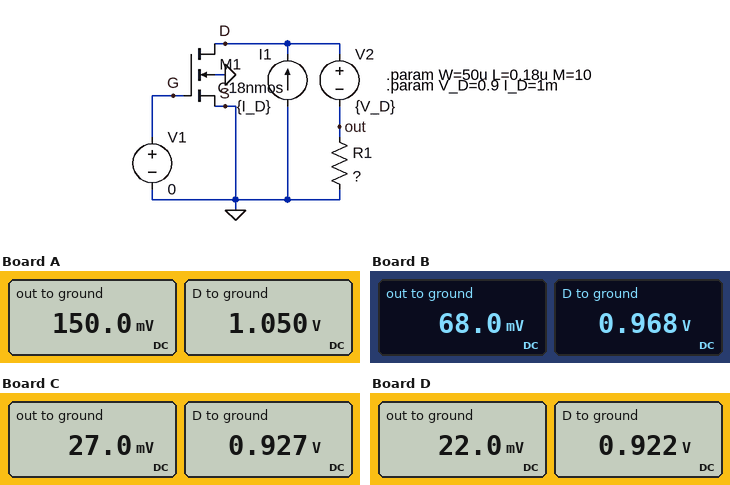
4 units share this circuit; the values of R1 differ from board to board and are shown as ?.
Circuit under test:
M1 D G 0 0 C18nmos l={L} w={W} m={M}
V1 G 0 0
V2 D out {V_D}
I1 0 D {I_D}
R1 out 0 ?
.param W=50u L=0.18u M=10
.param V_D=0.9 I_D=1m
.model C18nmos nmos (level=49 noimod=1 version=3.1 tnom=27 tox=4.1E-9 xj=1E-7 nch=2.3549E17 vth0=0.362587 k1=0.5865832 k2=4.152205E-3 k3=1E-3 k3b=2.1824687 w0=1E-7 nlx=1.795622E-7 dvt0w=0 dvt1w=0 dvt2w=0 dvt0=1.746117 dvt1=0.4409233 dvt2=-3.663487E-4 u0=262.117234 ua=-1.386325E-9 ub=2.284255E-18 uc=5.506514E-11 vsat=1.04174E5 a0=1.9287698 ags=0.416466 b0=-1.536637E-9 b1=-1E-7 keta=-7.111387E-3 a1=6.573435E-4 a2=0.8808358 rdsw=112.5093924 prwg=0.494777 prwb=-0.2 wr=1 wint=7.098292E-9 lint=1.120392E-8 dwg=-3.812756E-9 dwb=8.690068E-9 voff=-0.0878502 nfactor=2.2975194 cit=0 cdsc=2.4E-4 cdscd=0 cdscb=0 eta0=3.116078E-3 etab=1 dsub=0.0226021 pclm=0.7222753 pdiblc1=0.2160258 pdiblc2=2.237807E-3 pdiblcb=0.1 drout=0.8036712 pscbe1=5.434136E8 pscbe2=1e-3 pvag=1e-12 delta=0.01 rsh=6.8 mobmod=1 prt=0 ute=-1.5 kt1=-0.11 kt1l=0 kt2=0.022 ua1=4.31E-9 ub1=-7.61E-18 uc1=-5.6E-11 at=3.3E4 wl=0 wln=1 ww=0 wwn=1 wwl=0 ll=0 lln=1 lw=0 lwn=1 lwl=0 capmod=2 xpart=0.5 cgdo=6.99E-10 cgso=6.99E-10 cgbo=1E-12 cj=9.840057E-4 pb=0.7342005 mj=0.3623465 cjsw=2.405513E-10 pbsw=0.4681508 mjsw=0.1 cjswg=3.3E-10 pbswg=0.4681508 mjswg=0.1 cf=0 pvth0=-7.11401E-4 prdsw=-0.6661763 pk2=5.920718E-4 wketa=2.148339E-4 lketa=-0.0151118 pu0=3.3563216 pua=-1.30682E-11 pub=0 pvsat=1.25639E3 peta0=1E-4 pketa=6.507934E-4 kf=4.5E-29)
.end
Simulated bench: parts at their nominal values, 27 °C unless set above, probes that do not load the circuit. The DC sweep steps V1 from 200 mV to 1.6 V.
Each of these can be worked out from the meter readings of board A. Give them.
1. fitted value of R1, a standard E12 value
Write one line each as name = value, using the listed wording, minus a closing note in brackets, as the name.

fitted value of R1, a standard E12 value = 150 Ω
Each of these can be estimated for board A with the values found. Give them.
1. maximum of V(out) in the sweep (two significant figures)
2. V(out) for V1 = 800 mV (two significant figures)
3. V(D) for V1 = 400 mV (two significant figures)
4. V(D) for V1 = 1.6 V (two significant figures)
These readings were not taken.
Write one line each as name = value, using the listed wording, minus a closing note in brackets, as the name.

maximum of V(out) in the sweep = 150 mV
V(out) for V1 = 800 mV = -860 mV
V(D) for V1 = 400 mV = 1.0 V
V(D) for V1 = 1.6 V = 20 mV
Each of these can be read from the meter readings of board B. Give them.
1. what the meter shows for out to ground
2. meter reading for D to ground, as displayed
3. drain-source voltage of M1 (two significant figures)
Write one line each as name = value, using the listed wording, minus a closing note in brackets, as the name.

what the meter shows for out to ground = 68.0 mV
meter reading for D to ground, as displayed = 0.968 V
drain-source voltage of M1 = 970 mV
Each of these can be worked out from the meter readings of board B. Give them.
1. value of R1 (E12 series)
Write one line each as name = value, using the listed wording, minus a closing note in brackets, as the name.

value of R1 = 68 Ω
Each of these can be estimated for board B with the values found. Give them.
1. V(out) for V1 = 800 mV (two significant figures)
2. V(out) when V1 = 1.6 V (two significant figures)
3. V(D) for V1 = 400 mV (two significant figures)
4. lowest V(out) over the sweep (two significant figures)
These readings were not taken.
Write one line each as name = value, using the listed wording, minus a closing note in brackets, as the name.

V(out) for V1 = 800 mV = -820 mV
V(out) when V1 = 1.6 V = -860 mV
V(D) for V1 = 400 mV = 960 mV
lowest V(out) over the sweep = -860 mV
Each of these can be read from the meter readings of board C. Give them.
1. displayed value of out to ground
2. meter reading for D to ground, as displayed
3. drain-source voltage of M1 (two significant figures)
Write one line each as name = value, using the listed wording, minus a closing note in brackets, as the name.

displayed value of out to ground = 27.0 mV
meter reading for D to ground, as displayed = 0.927 V
drain-source voltage of M1 = 930 mV
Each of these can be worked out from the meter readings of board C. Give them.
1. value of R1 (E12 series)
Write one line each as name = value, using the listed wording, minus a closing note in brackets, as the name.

value of R1 = 27 Ω
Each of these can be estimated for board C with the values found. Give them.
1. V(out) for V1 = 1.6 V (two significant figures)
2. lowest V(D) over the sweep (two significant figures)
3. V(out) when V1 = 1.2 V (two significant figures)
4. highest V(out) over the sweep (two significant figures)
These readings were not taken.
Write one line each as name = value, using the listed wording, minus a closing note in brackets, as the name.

V(out) for V1 = 1.6 V = -810 mV
lowest V(D) over the sweep = 92 mV
V(out) when V1 = 1.2 V = -790 mV
highest V(out) over the sweep = 27 mV
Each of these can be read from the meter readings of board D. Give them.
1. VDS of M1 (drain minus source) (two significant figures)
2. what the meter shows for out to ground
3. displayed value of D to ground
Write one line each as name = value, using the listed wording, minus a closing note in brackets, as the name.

VDS of M1 (drain minus source) = 920 mV
what the meter shows for out to ground = 22.0 mV
displayed value of D to ground = 0.922 V
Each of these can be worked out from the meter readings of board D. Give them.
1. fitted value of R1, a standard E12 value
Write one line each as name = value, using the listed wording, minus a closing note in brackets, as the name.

fitted value of R1, a standard E12 value = 22 Ω
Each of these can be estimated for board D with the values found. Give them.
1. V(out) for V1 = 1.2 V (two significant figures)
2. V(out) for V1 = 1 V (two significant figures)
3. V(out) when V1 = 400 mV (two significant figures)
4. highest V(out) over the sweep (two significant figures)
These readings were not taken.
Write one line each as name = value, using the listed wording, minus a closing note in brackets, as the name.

V(out) for V1 = 1.2 V = -770 mV
V(out) for V1 = 1 V = -740 mV
V(out) when V1 = 400 mV = 19 mV
highest V(out) over the sweep = 22 mV
